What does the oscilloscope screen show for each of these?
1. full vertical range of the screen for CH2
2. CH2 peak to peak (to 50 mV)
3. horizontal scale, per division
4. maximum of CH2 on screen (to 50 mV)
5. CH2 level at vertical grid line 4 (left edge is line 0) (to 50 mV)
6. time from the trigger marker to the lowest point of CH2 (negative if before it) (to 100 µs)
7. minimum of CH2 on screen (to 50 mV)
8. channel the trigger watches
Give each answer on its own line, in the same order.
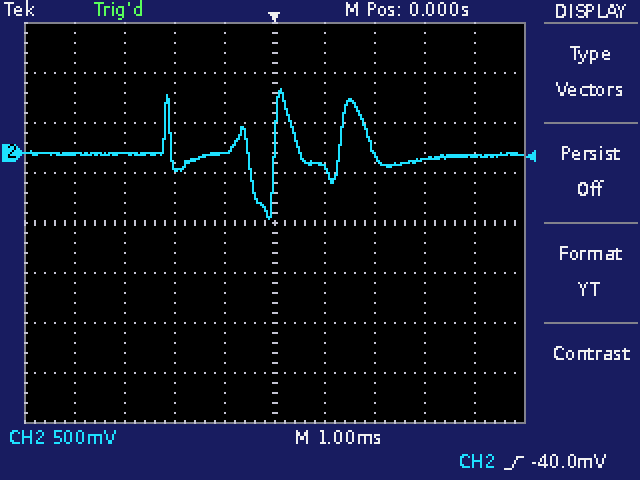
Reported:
4 V
1.30 V
1 ms
650 mV
0 mV
-100 µs
-650 mV
CH2
